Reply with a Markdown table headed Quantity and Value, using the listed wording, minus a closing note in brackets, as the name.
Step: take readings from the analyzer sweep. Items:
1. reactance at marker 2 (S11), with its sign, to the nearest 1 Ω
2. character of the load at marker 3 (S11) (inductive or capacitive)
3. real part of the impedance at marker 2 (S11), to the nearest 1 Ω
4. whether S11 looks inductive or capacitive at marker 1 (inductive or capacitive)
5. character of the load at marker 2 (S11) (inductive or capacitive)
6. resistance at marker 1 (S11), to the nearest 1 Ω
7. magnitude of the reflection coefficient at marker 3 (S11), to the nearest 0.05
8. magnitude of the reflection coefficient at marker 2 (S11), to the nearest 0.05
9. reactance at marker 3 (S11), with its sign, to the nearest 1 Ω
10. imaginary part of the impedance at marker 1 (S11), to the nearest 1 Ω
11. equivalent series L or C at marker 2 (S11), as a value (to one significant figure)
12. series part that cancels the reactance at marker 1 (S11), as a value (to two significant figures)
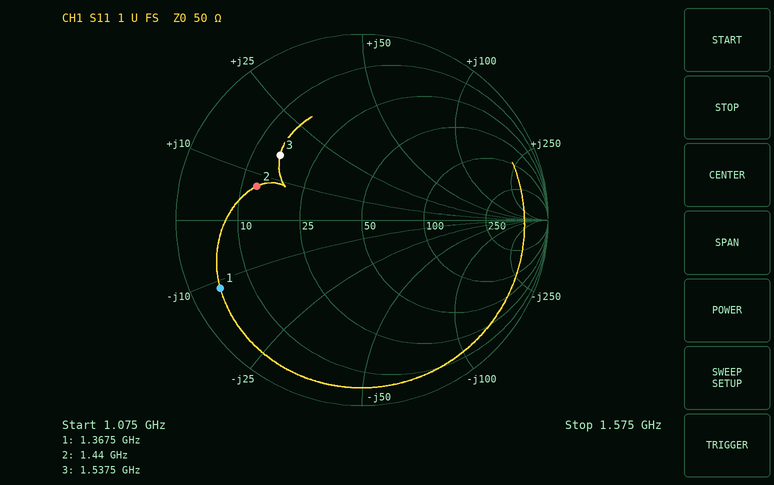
| Quantity | Value |
|---|---|
| reactance at marker 2 (S11), with its sign, to the nearest 1 Ω | +7 Ω |
| character of the load at marker 3 (S11) | inductive |
| real part of the impedance at marker 2 (S11), to the nearest 1 Ω | 13 Ω |
| whether S11 looks inductive or capacitive at marker 1 | capacitive |
| character of the load at marker 2 (S11) | inductive |
| resistance at marker 1 (S11), to the nearest 1 Ω | 4 Ω |
| magnitude of the reflection coefficient at marker 3 (S11), to the nearest 0.05 | 0.55 |
| magnitude of the reflection coefficient at marker 2 (S11), to the nearest 0.05 | 0.60 |
| reactance at marker 3 (S11), with its sign, to the nearest 1 Ω | +16 Ω |
| imaginary part of the impedance at marker 1 (S11), to the nearest 1 Ω | -11 Ω |
| equivalent series L or C at marker 2 (S11), as a value | 800 pH |
| series part that cancels the reactance at marker 1 (S11), as a value | 1.3 nH |
